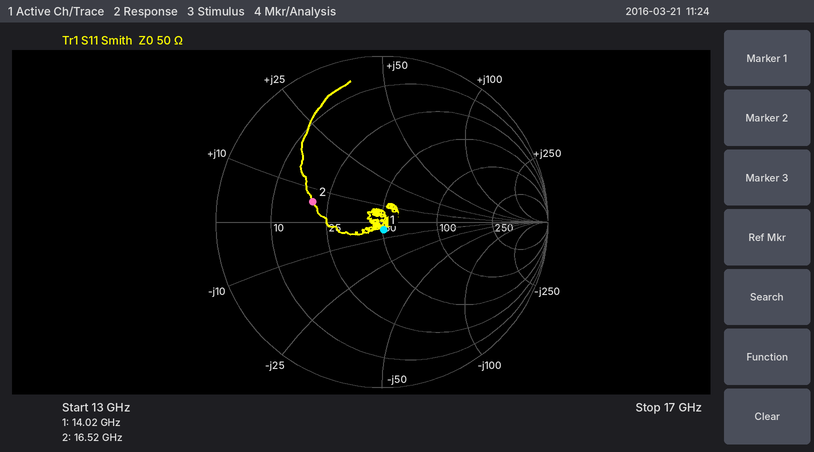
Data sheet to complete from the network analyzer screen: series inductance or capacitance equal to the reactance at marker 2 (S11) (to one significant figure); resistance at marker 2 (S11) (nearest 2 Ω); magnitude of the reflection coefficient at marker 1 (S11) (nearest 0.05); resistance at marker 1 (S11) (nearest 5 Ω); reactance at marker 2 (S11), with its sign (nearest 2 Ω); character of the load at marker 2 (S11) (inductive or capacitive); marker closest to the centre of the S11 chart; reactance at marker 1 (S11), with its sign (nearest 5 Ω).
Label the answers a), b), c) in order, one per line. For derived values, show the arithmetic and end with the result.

a) L = 6 Ω/(2π × 16.52 GHz) ≈ 57.8 pH, so 60 pH to one significant figure
b) 20 Ω
c) 0.05
d) 50 Ω
e) +6 Ω
f) inductive
g) marker 1
h) -5 Ω
